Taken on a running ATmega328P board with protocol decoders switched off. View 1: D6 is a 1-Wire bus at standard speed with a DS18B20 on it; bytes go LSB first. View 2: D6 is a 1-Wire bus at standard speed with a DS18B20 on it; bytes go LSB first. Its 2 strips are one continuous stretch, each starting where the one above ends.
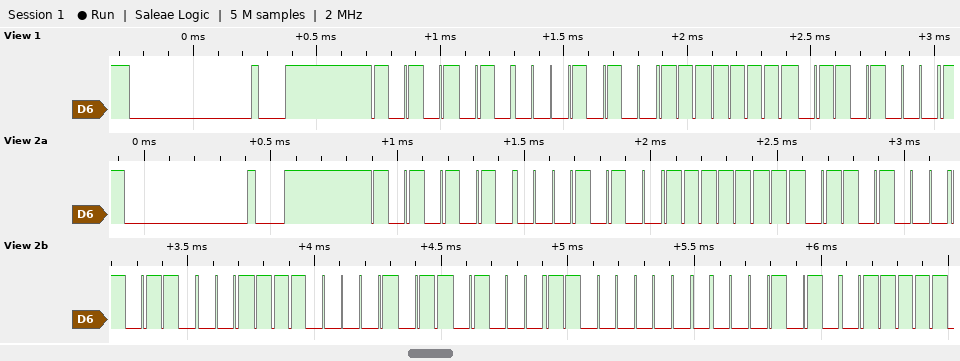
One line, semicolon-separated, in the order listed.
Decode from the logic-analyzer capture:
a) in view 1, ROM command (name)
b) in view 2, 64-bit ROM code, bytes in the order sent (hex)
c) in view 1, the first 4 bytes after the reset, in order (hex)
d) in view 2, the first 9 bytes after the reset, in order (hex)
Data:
Match ROM; 28 FF 16 8D 87 16 03 50; 55 28 FF 16; 55 28 FF 16 8D 87 16 03 50
